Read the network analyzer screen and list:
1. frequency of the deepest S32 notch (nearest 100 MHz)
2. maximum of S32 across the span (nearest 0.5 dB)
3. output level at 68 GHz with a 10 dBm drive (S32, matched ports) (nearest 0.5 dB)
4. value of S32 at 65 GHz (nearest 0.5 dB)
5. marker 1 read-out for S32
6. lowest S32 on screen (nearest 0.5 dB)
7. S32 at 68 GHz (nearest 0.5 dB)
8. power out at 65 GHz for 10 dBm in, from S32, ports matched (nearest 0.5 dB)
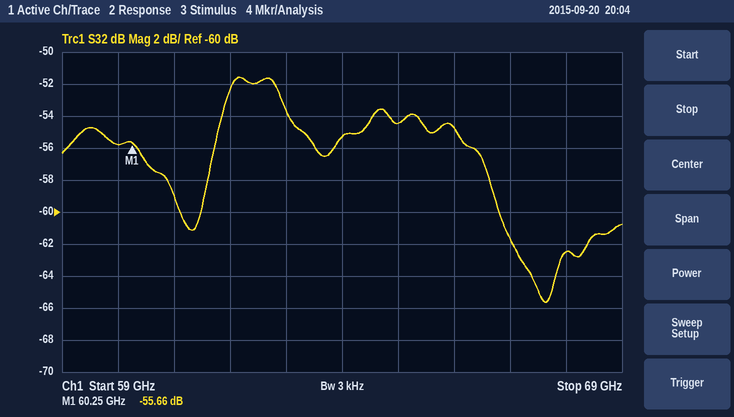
67.6 GHz
-51.5 dB
-52.5 dBm
-54.5 dB
-55.66 dB
-65.5 dB
-62.5 dB
-44.5 dBm
